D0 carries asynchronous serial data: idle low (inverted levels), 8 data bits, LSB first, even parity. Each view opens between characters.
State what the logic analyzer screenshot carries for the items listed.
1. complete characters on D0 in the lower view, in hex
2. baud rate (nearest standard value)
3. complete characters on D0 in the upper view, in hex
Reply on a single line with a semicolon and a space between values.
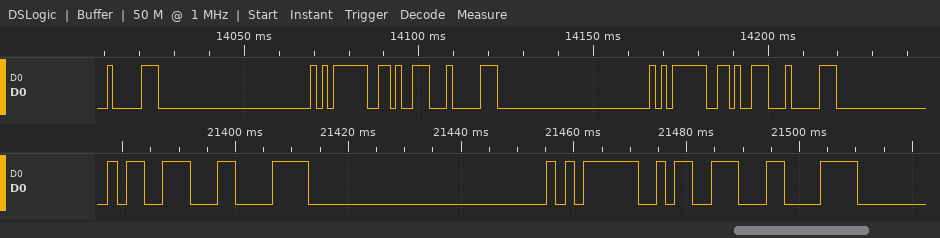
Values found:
19, 1E, 05, 19, 1E; 600 baud; 1F, 05, 1A, 1F, 05, 1A, 1F
